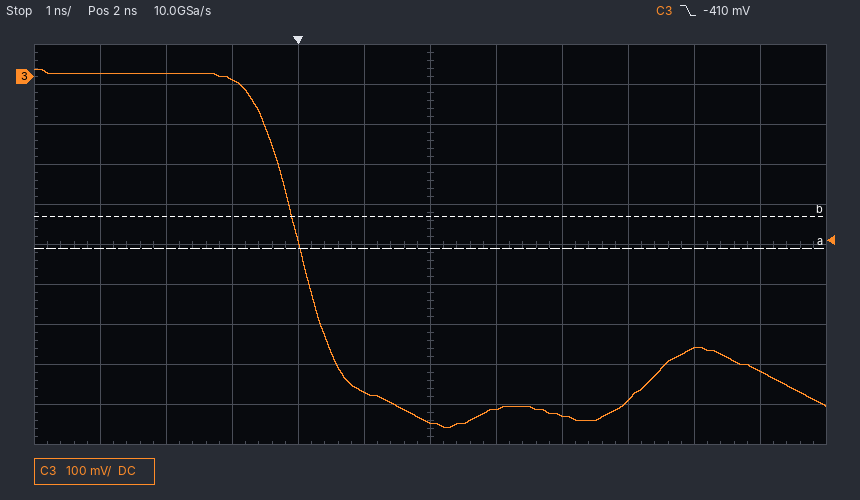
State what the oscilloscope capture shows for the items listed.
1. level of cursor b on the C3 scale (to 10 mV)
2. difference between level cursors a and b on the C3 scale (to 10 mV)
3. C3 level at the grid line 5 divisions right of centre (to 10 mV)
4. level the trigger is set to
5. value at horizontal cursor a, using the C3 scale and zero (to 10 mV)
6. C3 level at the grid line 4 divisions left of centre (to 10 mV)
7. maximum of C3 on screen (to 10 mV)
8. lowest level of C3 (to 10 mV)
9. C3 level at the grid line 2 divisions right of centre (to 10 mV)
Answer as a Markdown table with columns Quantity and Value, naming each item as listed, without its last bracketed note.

| Quantity | Value |
|---|---|
| level of cursor b on the C3 scale | -350 mV |
| difference between level cursors a and b on the C3 scale | 80 mV |
| C3 level at the grid line 5 divisions right of centre | -740 mV |
| level the trigger is set to | -410 mV |
| value at horizontal cursor a, using the C3 scale and zero | -430 mV |
| C3 level at the grid line 4 divisions left of centre | 10 mV |
| maximum of C3 on screen | 20 mV |
| lowest level of C3 | -880 mV |
| C3 level at the grid line 2 divisions right of centre | -850 mV |
